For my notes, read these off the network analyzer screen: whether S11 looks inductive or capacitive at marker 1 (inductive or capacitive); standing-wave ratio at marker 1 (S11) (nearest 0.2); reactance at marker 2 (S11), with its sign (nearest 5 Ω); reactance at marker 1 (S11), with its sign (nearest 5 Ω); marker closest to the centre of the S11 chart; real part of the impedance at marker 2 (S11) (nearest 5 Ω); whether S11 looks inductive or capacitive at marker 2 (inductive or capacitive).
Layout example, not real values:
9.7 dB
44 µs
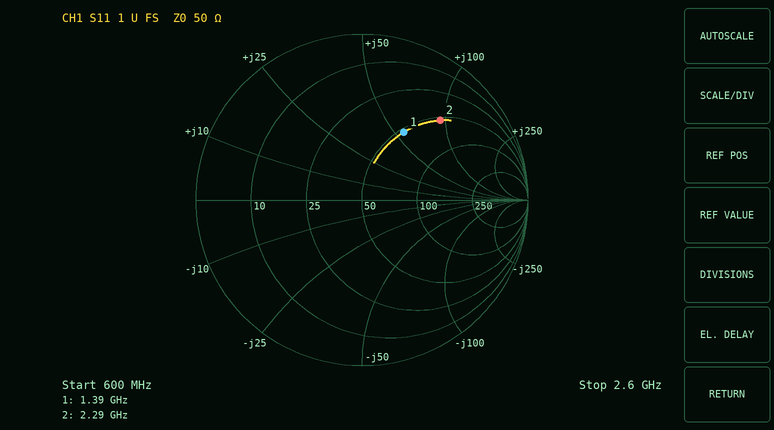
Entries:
inductive
2.8
+95 Ω
+55 Ω
marker 1
55 Ω
inductive
